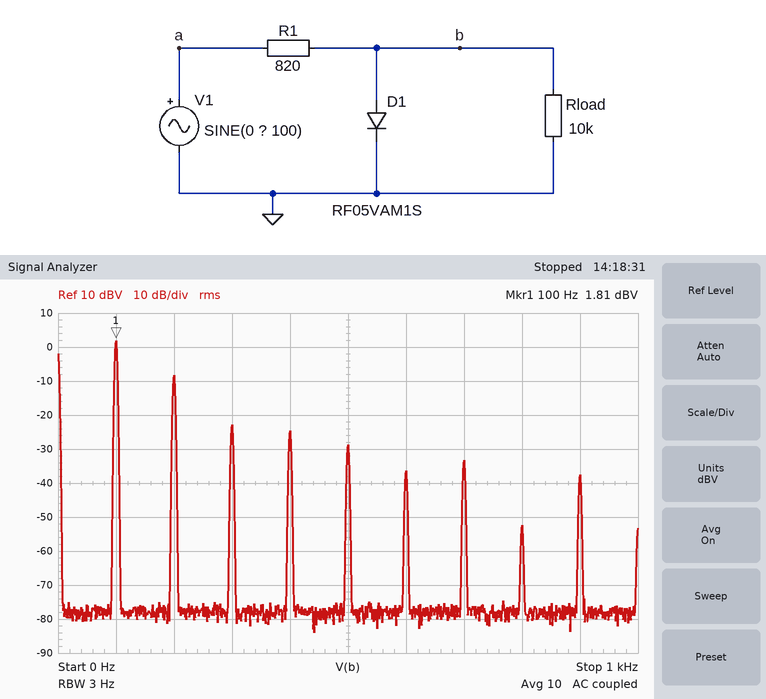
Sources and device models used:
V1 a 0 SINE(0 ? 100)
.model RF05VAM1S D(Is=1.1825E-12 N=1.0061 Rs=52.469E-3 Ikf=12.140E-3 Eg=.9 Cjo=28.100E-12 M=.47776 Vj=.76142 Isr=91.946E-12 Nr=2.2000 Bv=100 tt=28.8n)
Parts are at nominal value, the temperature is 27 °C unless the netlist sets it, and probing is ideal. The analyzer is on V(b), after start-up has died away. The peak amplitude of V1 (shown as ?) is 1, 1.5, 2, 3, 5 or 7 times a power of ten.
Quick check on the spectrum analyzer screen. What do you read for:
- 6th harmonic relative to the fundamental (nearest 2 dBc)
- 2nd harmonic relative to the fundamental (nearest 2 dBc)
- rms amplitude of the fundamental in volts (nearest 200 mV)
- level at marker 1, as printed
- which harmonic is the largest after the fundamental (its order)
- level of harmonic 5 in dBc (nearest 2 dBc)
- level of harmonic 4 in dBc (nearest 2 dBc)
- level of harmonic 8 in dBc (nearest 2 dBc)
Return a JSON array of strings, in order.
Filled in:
["-38 dBc", "-10 dBc", "1.2 V", "1.81 dBV", "2", "-30 dBc", "-26 dBc", "-54 dBc"]
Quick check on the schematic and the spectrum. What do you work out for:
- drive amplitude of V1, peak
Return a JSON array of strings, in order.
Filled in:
["3 V"]
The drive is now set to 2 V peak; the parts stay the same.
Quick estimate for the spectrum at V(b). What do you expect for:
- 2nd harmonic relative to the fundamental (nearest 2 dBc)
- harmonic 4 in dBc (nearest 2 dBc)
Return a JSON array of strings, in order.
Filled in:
["-12 dBc", "-32 dBc"]
